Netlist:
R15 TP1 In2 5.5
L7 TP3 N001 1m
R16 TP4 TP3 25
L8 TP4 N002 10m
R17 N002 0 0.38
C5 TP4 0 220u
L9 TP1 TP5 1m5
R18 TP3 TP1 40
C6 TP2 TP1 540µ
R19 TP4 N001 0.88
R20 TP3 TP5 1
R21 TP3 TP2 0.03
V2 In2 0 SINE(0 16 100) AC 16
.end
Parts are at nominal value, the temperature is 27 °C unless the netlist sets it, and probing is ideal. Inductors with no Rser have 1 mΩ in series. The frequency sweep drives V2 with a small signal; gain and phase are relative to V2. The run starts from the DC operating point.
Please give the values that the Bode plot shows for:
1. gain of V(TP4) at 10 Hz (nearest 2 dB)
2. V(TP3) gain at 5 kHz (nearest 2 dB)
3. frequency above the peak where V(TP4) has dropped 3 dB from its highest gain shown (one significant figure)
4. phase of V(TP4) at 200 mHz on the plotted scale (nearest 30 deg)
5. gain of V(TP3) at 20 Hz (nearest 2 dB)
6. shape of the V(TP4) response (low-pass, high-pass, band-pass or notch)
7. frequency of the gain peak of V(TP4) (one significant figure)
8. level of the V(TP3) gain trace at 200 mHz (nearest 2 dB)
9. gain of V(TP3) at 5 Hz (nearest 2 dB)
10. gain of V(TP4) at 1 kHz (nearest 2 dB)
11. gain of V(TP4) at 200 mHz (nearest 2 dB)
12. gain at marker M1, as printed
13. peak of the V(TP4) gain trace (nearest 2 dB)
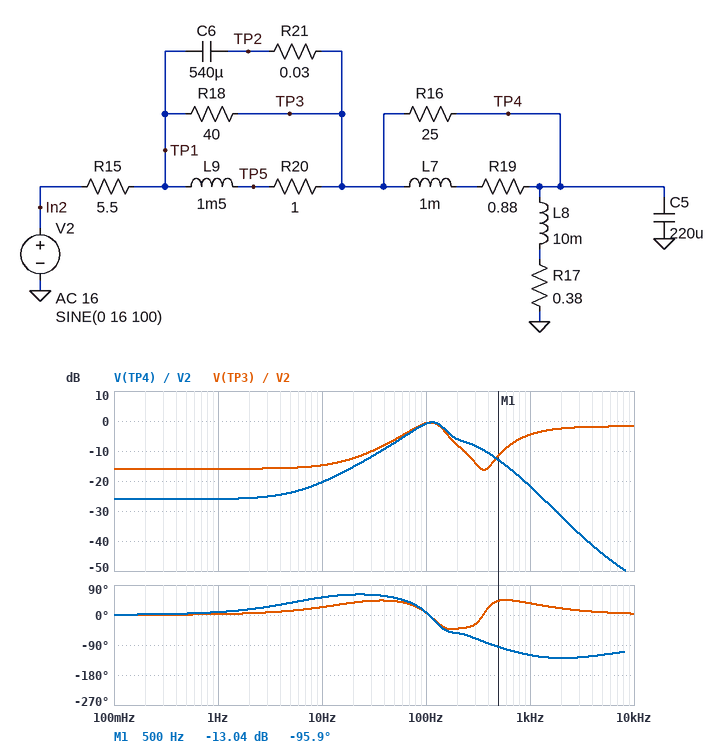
-20 dB
-2 dB
200 Hz
0 deg
-12 dB
band-pass
100 Hz
-16 dB
-16 dB
-22 dB
-26 dB
-13.04 dB
0 dB
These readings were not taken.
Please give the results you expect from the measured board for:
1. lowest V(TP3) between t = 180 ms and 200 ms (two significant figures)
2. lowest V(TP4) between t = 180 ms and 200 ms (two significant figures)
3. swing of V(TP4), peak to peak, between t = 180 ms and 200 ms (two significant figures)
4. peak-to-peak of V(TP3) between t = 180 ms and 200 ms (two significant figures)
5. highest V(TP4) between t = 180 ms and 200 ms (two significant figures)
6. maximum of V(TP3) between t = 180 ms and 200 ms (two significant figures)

-15 V
-14 V
29 V
29 V
14 V
15 V
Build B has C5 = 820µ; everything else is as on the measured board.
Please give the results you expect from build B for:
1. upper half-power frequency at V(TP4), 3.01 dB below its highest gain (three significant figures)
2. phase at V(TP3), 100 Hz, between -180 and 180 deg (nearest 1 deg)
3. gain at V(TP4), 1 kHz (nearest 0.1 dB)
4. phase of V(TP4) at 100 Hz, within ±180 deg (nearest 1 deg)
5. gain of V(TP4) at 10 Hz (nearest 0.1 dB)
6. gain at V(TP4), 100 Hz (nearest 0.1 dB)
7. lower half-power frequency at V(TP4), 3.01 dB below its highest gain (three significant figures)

75.9 Hz
-55 deg
-33.5 dB
-76 deg
-20.2 dB
-9.4 dB
43.8 Hz
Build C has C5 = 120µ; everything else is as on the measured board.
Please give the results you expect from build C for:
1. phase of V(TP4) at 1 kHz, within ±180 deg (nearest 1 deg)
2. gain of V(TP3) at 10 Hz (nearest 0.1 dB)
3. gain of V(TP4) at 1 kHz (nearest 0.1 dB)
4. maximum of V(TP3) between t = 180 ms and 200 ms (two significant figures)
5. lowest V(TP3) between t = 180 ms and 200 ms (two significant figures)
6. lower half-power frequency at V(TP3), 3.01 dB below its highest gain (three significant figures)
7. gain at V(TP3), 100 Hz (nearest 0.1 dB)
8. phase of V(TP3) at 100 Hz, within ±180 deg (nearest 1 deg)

-117 deg
-14.8 dB
-16.1 dB
13 V
-13 V
82.3 Hz
-2.0 dB
26 deg
